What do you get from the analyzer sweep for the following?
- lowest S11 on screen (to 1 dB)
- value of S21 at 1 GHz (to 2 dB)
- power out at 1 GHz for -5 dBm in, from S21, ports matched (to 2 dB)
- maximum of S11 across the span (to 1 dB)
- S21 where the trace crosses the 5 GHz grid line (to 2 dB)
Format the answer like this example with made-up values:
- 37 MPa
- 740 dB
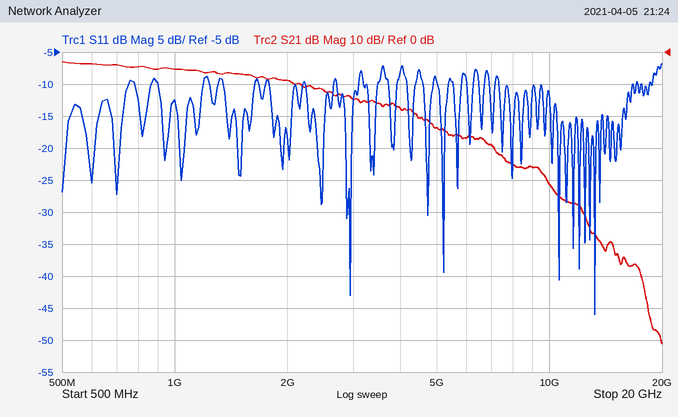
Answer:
- -46 dB
- -6 dB
- -10 dBm
- -7 dB
- -24 dB
